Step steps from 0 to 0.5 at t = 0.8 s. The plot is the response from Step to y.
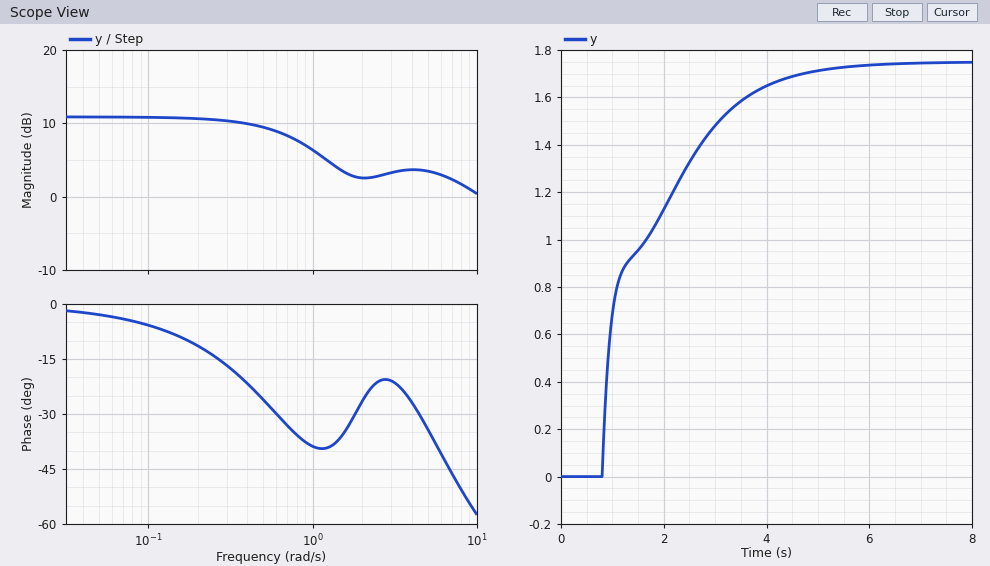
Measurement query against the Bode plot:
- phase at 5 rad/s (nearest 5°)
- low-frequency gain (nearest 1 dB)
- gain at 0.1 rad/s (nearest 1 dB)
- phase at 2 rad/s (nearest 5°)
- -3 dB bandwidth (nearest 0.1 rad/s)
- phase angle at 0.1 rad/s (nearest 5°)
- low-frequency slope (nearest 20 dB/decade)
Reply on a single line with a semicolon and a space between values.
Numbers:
-35°; 11 dB; 11 dB; -25°; 0.8 rad/s; -5°; 0 dB/decade
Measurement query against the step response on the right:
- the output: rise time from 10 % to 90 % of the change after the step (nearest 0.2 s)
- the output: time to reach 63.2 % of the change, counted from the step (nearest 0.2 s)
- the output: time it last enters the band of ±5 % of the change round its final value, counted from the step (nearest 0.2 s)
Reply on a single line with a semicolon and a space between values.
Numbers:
2.6 s; 1.2 s; 3.4 s
